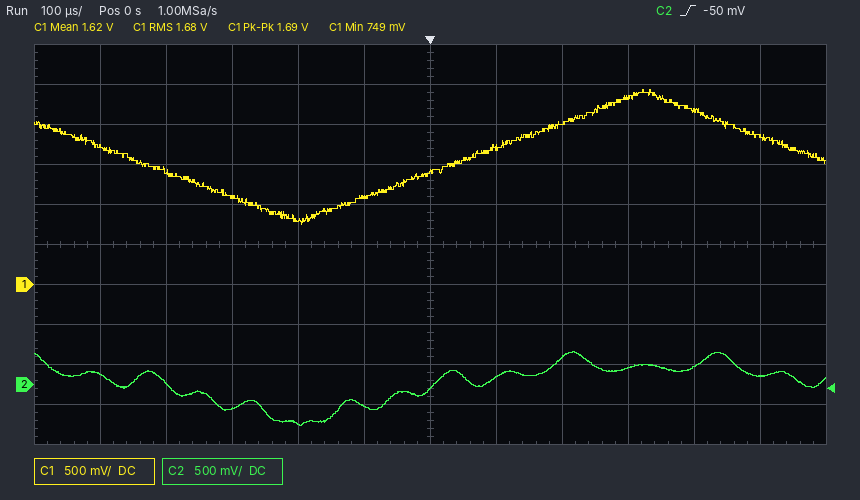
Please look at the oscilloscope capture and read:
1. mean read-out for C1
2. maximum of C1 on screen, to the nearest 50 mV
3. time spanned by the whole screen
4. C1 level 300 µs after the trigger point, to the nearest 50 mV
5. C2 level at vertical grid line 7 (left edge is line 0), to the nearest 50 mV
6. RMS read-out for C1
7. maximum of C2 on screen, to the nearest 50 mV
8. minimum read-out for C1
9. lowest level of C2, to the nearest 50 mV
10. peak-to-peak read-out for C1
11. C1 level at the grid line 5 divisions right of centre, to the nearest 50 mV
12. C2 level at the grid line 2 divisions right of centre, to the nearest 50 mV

1.62 V
2.45 V
1.2 ms
2.35 V
100 mV
1.68 V
400 mV
749 mV
-500 mV
1.69 V
1.85 V
350 mV
